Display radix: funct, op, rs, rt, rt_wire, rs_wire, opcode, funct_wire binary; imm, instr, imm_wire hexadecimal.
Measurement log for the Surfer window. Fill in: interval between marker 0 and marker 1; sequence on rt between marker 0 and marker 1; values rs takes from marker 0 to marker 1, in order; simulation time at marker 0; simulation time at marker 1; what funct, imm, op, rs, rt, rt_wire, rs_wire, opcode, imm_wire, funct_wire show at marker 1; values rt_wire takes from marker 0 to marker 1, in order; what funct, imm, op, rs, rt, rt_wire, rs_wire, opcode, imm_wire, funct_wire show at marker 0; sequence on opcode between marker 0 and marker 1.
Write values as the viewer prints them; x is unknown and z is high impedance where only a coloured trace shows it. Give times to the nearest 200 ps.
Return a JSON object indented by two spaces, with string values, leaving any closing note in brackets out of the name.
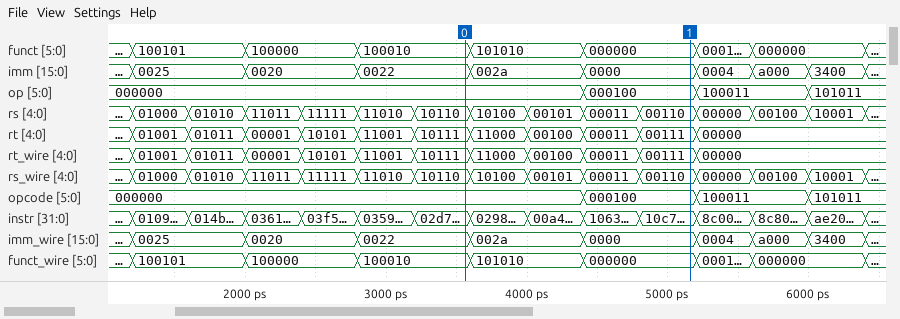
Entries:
{
  "interval between marker 0 and marker 1": "1600 ps",
  "sequence on rt between marker 0 and marker 1": "10111, 11000, 00100, 00011, 00111",
  "values rs takes from marker 0 to marker 1, in order": "10110, 10100, 00101, 00011, 00110",
  "simulation time at marker 0": "3600 ps",
  "simulation time at marker 1": "5200 ps",
  "what funct, imm, op, rs, rt, rt_wire, rs_wire, opcode, imm_wire, funct_wire show at marker 1": "funct=000000, imm=0000, op=000100, rs=00110, rt=00111, rt_wire=00111, rs_wire=00110, opcode=000100, imm_wire=0000, funct_wire=000000",
  "values rt_wire takes from marker 0 to marker 1, in order": "10111, 11000, 00100, 00011, 00111",
  "what funct, imm, op, rs, rt, rt_wire, rs_wire, opcode, imm_wire, funct_wire show at marker 0": "funct=100010, imm=0022, op=000000, rs=10110, rt=10111, rt_wire=10111, rs_wire=10110, opcode=000000, imm_wire=0022, funct_wire=100010",
  "sequence on opcode between marker 0 and marker 1": "000000, 000100"
}
